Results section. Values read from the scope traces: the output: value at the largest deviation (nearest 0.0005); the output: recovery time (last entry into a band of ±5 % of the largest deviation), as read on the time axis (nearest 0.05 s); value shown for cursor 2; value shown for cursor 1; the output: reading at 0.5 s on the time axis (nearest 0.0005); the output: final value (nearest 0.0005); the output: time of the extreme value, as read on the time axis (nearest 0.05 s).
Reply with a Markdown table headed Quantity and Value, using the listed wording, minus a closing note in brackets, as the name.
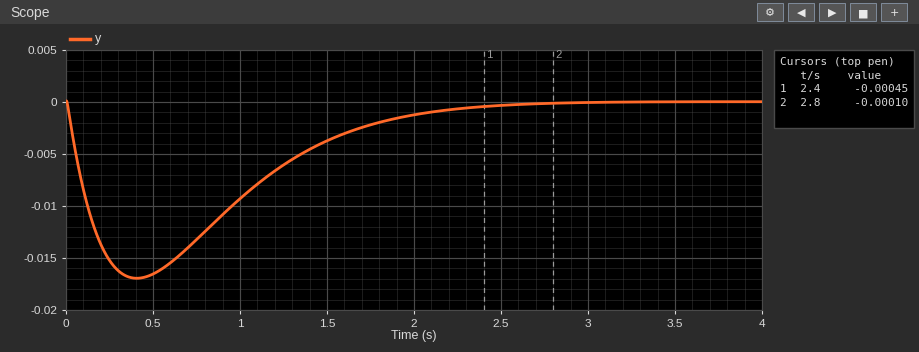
| Quantity | Value |
|---|---|
| the output: value at the largest deviation | -0.0170 |
| the output: recovery time (last entry into a band of ±5 % of the largest deviation), as read on the time axis | 2.15 s |
| value shown for cursor 2 | -0.00010 |
| value shown for cursor 1 | -0.00045 |
| the output: reading at 0.5 s on the time axis | -0.0165 |
| the output: final value | 0.0000 |
| the output: time of the extreme value, as read on the time axis | 0.40 s |
